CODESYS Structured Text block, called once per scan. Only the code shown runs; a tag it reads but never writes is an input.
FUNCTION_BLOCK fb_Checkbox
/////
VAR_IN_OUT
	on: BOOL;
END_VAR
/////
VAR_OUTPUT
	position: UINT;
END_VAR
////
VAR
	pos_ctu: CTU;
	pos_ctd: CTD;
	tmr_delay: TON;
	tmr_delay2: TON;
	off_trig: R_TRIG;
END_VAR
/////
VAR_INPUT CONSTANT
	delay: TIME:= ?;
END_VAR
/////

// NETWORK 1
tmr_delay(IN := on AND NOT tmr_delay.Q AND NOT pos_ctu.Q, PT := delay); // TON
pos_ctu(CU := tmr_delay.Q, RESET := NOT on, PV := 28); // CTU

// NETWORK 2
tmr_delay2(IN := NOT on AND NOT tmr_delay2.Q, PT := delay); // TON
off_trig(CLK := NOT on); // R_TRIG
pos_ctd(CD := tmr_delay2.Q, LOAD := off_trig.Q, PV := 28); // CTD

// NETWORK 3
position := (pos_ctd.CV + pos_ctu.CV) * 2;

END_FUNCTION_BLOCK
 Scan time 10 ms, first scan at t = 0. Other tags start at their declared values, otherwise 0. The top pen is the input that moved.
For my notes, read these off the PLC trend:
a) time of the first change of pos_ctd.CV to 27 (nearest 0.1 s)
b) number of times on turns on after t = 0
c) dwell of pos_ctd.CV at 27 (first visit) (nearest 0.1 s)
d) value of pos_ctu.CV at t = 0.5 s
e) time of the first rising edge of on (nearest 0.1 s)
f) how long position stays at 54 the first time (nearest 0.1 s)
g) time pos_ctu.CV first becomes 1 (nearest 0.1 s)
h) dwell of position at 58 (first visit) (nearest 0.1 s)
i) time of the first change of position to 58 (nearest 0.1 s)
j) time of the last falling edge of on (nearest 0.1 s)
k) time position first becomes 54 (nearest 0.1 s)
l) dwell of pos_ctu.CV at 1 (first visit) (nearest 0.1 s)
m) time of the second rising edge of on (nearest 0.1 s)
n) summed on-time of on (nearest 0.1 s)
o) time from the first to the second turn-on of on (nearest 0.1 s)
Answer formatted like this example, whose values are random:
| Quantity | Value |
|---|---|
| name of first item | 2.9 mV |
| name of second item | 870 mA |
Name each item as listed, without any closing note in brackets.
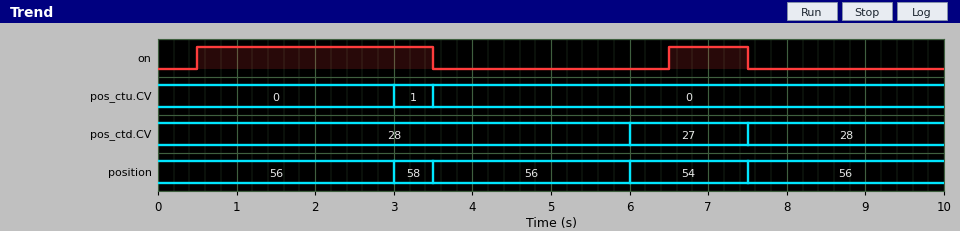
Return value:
| Quantity | Value |
|---|---|
| time of the first change of pos_ctd.CV to 27 | 6.0 s |
| number of times on turns on after t = 0 | 2 |
| dwell of pos_ctd.CV at 27 (first visit) | 1.5 s |
| value of pos_ctu.CV at t = 0.5 s | 0 |
| time of the first rising edge of on | 0.5 s |
| how long position stays at 54 the first time | 1.5 s |
| time pos_ctu.CV first becomes 1 | 3.0 s |
| dwell of position at 58 (first visit) | 0.5 s |
| time of the first change of position to 58 | 3.0 s |
| time of the last falling edge of on | 7.5 s |
| time position first becomes 54 | 6.0 s |
| dwell of pos_ctu.CV at 1 (first visit) | 0.5 s |
| time of the second rising edge of on | 6.5 s |
| summed on-time of on | 4.0 s |
| time from the first to the second turn-on of on | 6.0 s |
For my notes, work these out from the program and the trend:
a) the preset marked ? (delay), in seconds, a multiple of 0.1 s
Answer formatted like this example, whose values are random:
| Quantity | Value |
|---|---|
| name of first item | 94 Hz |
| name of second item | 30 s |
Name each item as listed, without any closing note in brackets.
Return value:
| Quantity | Value |
|---|---|
| the preset marked ? (delay), in seconds, a multiple of 0.1 s | 2.5 s |
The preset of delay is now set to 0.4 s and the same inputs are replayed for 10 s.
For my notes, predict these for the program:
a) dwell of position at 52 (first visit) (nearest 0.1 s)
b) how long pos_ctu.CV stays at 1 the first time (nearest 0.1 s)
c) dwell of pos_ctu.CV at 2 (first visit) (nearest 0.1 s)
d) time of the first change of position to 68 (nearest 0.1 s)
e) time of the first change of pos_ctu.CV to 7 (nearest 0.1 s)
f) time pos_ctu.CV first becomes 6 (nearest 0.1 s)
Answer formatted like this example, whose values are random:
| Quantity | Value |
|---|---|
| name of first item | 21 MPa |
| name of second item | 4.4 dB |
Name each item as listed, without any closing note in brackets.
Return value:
| Quantity | Value |
|---|---|
| dwell of position at 52 (first visit) | 0.4 s |
| how long pos_ctu.CV stays at 1 the first time | 0.4 s |
| dwell of pos_ctu.CV at 2 (first visit) | 0.4 s |
| time of the first change of position to 68 | 3.4 s |
| time of the first change of pos_ctu.CV to 7 | 3.4 s |
| time pos_ctu.CV first becomes 6 | 3.0 s |
